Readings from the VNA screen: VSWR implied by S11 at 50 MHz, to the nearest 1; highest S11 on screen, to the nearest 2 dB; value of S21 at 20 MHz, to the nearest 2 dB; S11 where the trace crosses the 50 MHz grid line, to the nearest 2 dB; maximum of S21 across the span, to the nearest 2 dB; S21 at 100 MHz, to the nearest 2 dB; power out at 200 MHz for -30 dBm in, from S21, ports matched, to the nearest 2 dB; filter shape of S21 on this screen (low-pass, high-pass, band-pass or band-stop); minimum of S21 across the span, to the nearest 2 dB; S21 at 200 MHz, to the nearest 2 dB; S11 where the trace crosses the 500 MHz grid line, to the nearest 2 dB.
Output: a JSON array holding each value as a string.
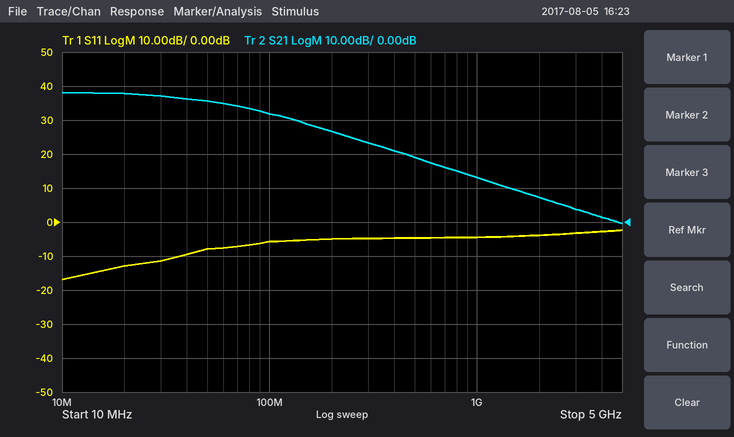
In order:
["2", "-2 dB", "38 dB", "-8 dB", "38 dB", "32 dB", "-4 dBm", "low-pass", "0 dB", "26 dB", "-4 dB"]
